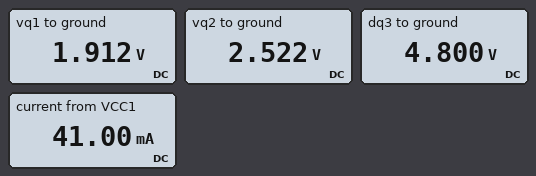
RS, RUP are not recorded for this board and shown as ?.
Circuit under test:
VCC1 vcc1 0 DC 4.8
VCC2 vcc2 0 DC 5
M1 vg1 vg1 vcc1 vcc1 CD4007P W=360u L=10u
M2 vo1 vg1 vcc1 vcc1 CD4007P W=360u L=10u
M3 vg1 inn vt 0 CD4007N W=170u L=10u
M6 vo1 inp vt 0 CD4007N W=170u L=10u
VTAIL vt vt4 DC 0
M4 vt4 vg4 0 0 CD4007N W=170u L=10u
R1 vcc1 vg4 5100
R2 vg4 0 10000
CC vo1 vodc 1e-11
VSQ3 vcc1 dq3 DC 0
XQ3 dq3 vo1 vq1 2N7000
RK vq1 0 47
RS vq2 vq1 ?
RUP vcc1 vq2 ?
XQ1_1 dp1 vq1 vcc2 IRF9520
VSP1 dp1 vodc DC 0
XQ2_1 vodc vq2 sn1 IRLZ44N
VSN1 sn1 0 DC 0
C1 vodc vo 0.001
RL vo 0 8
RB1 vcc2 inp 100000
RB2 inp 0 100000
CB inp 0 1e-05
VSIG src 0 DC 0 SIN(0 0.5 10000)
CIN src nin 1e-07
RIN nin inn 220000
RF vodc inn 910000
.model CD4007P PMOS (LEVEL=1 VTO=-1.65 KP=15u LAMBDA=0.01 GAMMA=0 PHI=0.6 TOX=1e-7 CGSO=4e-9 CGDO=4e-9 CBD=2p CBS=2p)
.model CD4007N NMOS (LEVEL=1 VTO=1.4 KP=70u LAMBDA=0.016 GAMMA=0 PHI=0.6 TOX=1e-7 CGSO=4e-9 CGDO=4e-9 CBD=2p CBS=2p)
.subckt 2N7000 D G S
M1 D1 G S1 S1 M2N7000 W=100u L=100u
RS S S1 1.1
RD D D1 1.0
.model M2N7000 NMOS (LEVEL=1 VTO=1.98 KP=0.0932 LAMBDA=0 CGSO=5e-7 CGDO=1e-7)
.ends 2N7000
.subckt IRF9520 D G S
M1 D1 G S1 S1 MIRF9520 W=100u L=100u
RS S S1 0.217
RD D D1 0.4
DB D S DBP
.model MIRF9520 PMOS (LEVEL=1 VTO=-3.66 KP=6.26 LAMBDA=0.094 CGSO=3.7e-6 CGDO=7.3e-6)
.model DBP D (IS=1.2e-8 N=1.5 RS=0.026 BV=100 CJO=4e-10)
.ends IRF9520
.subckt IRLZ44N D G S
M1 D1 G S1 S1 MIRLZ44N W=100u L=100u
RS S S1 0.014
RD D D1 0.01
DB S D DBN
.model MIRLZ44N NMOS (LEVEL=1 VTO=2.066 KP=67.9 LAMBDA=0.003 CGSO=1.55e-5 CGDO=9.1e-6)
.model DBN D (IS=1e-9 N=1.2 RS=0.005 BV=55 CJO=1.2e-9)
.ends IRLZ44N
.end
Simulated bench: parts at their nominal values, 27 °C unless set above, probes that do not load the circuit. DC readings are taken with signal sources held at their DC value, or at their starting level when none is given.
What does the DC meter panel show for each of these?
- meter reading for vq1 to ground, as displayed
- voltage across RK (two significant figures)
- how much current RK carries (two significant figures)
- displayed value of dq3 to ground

1.912 V
1.9 V
41 mA
4.800 V
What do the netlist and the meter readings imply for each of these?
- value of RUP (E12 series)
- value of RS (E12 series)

56 Ω
15 Ω
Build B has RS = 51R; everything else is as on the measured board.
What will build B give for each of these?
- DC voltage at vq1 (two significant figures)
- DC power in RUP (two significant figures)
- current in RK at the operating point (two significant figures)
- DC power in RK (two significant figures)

1.5 V
54 mW
31 mA
46 mW
